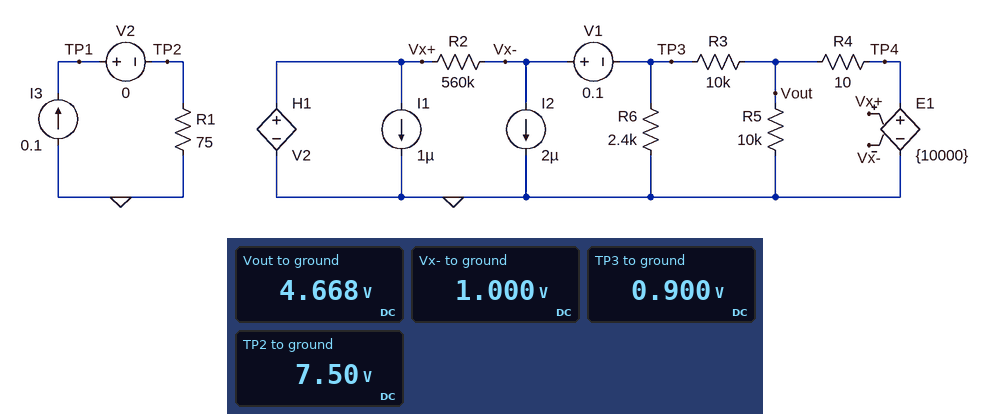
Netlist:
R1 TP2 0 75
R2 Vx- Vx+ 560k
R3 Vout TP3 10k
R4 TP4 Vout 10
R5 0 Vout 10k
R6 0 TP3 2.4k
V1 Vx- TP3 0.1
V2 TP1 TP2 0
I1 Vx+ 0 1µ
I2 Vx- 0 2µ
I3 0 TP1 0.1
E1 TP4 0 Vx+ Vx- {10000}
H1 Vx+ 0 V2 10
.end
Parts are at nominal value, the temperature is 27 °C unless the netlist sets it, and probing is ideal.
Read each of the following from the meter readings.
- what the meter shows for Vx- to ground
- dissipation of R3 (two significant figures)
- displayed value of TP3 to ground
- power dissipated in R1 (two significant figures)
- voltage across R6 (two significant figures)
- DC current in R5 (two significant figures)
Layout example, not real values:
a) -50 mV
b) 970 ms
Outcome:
a) 1.000 V
b) 1.4 mW
c) 0.900 V
d) 750 mW
e) 900 mV
f) 470 µA
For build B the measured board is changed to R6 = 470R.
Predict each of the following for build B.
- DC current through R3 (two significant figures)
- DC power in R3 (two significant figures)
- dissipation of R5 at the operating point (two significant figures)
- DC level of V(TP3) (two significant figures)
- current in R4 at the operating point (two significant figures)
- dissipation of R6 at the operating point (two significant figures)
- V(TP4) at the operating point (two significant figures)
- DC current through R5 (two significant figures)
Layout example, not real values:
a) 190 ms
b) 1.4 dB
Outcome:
a) 1.9 mA
b) 37 mW
c) 40 mW
d) 900 mV
e) 3.9 mA
f) 1.7 mW
g) 20 V
h) 2.0 mA
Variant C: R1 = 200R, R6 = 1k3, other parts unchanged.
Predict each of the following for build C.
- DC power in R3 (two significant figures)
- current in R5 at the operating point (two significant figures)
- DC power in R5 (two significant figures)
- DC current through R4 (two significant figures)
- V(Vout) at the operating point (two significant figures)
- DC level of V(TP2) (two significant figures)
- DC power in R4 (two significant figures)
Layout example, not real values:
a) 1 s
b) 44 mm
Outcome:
a) 4.8 mW
b) 780 µA
c) 6.1 mW
d) 1.5 mA
e) 7.8 V
f) 20 V
g) 22 µW
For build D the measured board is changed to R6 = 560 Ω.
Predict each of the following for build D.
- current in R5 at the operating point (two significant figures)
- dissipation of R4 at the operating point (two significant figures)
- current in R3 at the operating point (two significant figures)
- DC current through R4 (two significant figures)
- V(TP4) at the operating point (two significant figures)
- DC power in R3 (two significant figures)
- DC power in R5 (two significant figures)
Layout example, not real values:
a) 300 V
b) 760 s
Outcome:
a) 1.7 mA
b) 110 µW
c) 1.6 mA
d) 3.3 mA
e) 17 V
f) 26 mW
g) 29 mW
